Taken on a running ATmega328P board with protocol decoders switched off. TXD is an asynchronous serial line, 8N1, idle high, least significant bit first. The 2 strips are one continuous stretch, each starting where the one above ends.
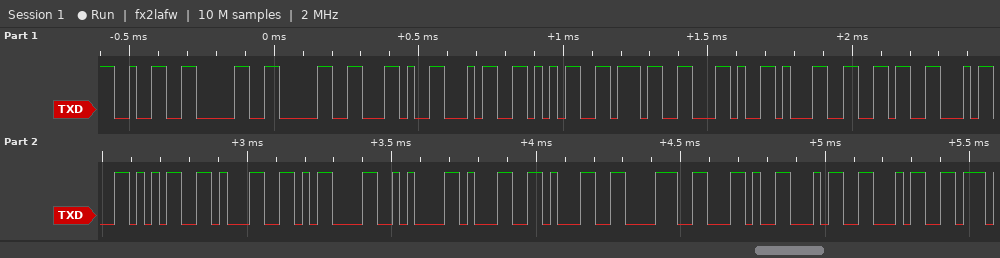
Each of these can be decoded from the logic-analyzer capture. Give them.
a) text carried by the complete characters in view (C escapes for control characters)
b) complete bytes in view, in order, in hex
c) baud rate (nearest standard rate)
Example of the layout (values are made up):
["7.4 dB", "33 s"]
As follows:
["\"200,457,16451\\r\\n118,44\"", "32 30 30 2C 34 35 37 2C 31 36 34 35 31 0D 0A 31 31 38 2C 34 34", "38400 baud"]
